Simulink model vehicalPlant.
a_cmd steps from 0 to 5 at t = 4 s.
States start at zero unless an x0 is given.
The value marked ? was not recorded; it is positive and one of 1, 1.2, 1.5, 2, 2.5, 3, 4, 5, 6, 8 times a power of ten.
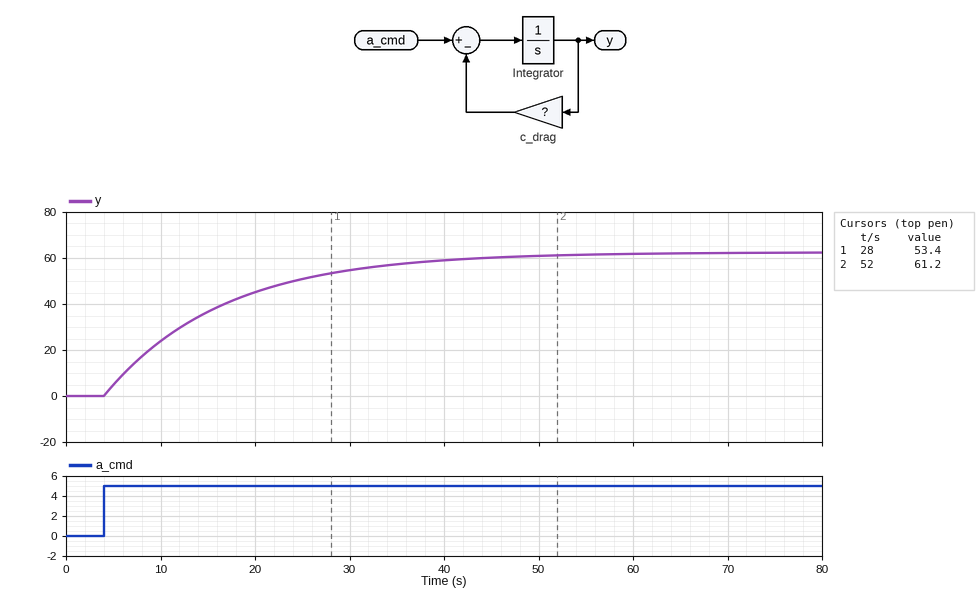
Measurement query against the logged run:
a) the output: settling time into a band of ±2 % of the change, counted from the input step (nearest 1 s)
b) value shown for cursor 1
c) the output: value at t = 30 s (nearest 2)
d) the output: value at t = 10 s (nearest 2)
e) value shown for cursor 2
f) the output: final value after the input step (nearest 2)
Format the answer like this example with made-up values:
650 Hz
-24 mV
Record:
49 s
53.4
54
24
61.2
62
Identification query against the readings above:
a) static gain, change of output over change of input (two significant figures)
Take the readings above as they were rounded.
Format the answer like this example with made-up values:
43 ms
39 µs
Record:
12
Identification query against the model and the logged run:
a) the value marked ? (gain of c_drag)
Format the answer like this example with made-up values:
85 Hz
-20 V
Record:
0.08
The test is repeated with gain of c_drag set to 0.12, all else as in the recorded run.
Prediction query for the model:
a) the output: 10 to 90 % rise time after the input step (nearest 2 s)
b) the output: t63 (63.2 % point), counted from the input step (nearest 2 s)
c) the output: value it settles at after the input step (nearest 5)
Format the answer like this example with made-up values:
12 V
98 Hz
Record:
18 s
8 s
40
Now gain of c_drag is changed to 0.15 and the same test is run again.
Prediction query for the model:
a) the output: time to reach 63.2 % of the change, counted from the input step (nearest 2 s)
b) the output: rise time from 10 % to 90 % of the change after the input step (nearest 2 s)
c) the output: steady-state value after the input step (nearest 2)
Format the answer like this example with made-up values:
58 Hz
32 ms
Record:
6 s
14 s
34
